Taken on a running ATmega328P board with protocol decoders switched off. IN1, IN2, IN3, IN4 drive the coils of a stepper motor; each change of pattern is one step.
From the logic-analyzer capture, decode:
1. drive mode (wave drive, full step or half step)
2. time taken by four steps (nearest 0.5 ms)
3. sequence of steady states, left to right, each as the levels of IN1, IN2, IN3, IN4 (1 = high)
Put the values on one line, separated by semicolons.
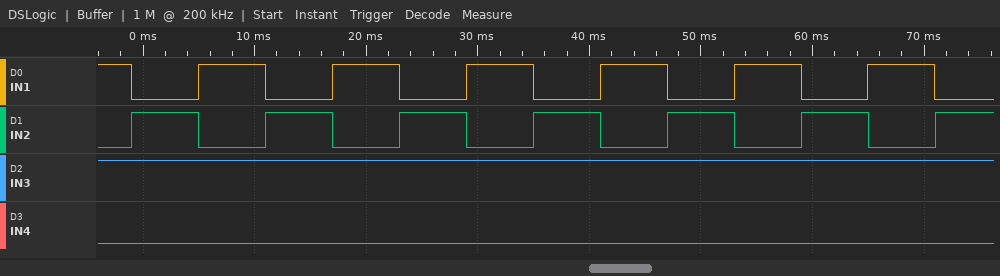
full step; 24.0 ms; 1010 0110 1010 0110 1010 0110 1010 0110 1010 0110 1010 0110 1010 0110
